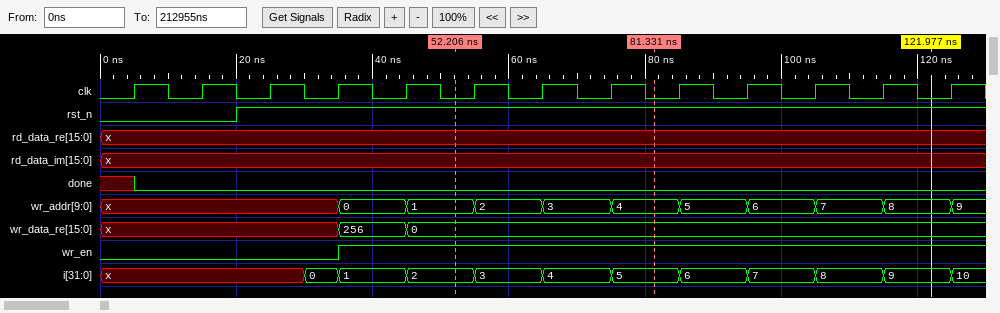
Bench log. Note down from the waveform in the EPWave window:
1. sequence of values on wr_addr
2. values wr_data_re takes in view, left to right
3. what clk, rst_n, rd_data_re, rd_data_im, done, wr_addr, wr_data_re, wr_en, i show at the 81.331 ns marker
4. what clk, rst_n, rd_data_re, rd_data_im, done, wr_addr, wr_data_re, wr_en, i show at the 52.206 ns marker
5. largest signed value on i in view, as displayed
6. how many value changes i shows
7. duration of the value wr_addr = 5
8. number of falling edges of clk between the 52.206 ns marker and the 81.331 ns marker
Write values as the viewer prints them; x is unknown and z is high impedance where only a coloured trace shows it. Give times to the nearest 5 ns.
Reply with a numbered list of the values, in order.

1. x, 0, 1, 2, 3, 4, 5, 6, 7, 8, 9
2. x, 256, 0
3. clk=0, rst_n=1, rd_data_re=x, rd_data_im=x, done=0, wr_addr=4, wr_data_re=0, wr_en=1, i=5
4. clk=0, rst_n=1, rd_data_re=x, rd_data_im=x, done=0, wr_addr=1, wr_data_re=0, wr_en=1, i=2
5. 10
6. 11
7. 10 ns
8. 3
